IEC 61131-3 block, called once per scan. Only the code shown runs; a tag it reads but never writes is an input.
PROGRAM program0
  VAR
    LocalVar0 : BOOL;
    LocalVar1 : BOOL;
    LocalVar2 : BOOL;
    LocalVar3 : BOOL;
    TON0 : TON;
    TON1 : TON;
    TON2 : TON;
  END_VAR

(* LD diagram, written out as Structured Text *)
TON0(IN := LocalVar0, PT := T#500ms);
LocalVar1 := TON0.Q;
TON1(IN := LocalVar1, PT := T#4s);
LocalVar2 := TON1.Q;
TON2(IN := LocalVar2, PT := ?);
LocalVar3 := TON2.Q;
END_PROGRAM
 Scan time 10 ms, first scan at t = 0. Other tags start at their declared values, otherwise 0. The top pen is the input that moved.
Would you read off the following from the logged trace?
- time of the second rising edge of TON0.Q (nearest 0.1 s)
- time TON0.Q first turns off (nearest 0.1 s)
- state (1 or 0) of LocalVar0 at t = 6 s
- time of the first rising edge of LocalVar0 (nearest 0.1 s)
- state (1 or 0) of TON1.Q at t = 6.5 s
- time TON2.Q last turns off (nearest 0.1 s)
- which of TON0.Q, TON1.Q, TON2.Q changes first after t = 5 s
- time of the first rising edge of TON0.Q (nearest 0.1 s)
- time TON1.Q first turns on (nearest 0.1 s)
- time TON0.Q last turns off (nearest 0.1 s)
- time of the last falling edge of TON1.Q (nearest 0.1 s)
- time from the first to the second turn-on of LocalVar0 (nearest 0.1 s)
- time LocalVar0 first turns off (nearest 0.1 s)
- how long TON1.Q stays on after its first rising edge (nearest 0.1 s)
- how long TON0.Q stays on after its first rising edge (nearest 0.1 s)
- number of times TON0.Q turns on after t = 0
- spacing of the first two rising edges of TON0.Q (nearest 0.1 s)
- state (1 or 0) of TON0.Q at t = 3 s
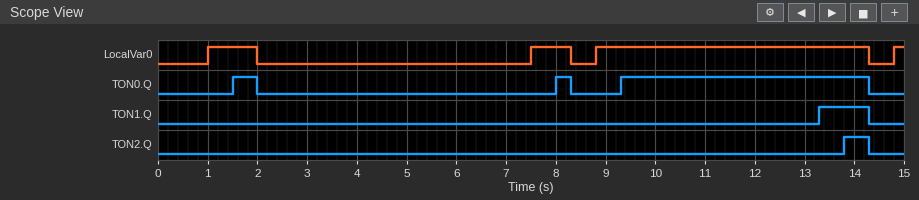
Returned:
8.0 s
2.0 s
0
1.0 s
0
14.3 s
TON0.Q
1.5 s
13.3 s
14.3 s
14.3 s
6.5 s
2.0 s
1.0 s
0.5 s
3
6.5 s
0
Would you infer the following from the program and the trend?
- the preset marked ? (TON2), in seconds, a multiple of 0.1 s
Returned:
0.5 s
